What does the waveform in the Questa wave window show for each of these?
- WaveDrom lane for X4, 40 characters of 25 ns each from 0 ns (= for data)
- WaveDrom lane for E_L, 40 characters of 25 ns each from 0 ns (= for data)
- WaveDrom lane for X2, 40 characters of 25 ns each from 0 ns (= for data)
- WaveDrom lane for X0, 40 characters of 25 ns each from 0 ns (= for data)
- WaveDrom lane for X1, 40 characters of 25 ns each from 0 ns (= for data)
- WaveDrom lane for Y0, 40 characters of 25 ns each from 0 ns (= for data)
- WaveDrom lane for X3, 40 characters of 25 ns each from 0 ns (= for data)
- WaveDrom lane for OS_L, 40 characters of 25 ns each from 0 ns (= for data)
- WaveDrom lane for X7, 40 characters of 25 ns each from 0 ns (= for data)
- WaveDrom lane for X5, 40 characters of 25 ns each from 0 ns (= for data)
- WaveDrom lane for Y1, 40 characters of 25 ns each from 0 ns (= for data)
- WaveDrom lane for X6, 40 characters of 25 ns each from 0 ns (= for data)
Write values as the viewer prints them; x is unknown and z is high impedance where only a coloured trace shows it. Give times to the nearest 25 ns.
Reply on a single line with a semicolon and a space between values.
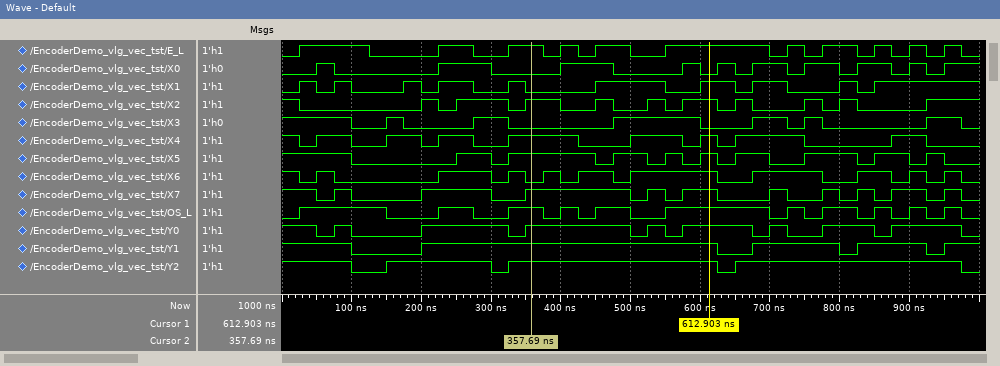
{name: 'X4', wave: '101.0.1.01.0.1...0..1..0101...0....1.0..'}; {name: 'E_L', wave: '01...0...1.0.1.0101.0.1.....0101.0101010'}; {name: 'X2', wave: '10......101..01.0.10.101.010..1010...1..'}; {name: 'X0', wave: '0.10.....1..0...1..0...10101.01.01.0101.'}; {name: 'X1', wave: '01010..101.0.10...1...0.1.01.0..101.....'}; {name: 'Y0', wave: '1.010...1....01.....0101...010.1..01...0'}; {name: 'X3', wave: '1...0.10...1.0.....1....0..1.010.....1.0'}; {name: 'OS_L', wave: '01....0..1.0.1.0101.0.1.....0101.0101010'}; {name: 'X7', wave: '1.010...1...0.1.....0101.0..10.10101.010'}; {name: 'X5', wave: '1...0.....1.01....01.010101.0.1..01.010.'}; {name: 'Y1', wave: '1...0...1................0.1....01...01.'}; {name: 'X6', wave: '1010.....1..010101.01....0.1...0.1.01010'}
